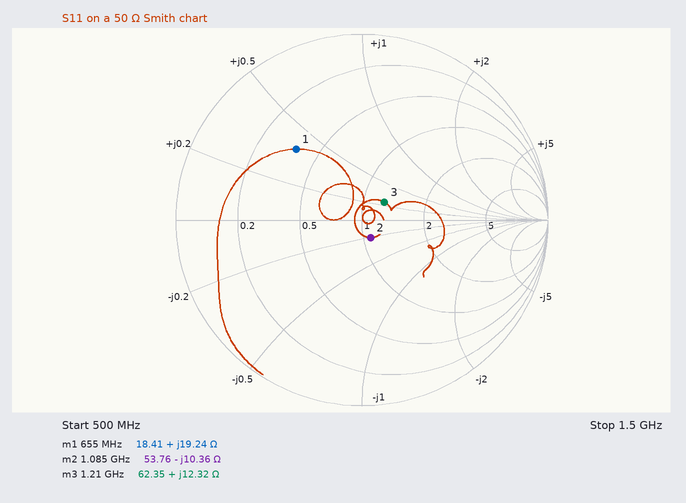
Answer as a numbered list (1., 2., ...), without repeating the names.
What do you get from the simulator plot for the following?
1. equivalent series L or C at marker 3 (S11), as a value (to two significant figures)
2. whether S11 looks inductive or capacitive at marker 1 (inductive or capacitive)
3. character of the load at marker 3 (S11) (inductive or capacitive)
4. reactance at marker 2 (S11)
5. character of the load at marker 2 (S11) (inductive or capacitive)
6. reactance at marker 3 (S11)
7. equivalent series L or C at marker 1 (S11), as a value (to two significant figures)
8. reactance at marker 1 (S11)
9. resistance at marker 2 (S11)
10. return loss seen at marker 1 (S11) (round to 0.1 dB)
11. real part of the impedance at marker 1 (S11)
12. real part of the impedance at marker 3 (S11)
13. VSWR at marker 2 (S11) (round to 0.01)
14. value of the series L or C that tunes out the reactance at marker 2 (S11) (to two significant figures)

1. 1.6 nH
2. inductive
3. inductive
4. -10.36 Ω
5. capacitive
6. +12.32 Ω
7. 4.7 nH
8. +19.24 Ω
9. 53.76 Ω
10. 5.7 dB
11. 18.41 Ω
12. 62.35 Ω
13. 1.24
14. 1.5 nH
